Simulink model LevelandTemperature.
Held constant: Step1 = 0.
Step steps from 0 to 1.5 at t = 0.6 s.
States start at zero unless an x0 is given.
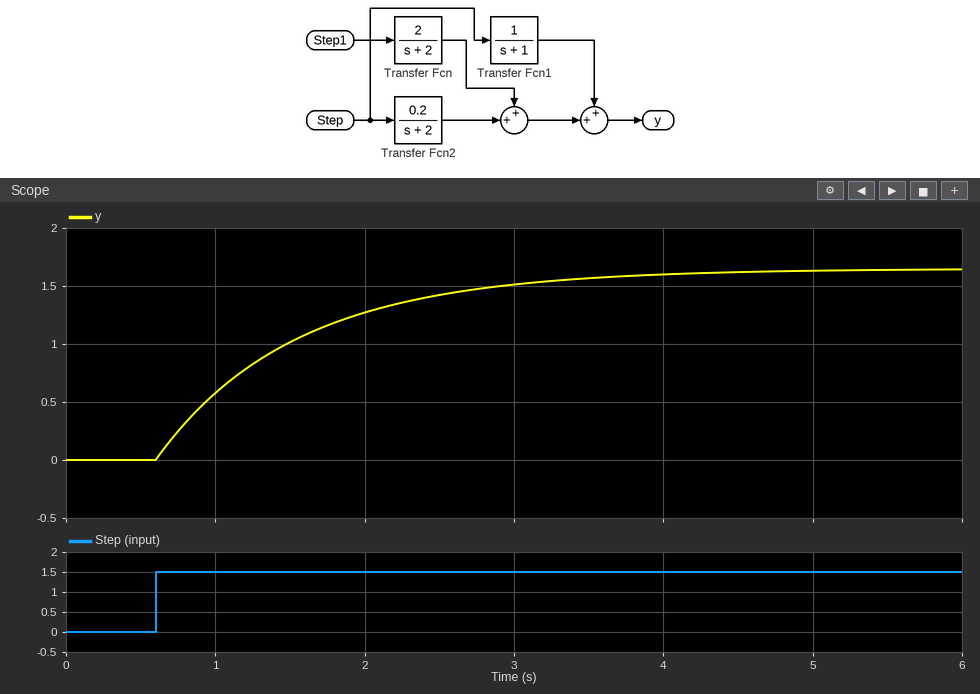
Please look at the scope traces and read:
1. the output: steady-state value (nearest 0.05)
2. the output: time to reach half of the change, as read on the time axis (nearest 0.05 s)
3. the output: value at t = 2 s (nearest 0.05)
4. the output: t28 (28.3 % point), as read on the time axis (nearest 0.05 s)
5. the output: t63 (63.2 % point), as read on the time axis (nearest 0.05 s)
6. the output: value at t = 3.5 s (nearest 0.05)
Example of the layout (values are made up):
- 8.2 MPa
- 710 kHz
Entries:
- 1.65
- 1.25 s
- 1.25
- 0.90 s
- 1.55 s
- 1.55
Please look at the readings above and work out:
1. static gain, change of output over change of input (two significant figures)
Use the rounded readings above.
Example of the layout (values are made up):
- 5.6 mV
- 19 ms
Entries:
- 1.1
